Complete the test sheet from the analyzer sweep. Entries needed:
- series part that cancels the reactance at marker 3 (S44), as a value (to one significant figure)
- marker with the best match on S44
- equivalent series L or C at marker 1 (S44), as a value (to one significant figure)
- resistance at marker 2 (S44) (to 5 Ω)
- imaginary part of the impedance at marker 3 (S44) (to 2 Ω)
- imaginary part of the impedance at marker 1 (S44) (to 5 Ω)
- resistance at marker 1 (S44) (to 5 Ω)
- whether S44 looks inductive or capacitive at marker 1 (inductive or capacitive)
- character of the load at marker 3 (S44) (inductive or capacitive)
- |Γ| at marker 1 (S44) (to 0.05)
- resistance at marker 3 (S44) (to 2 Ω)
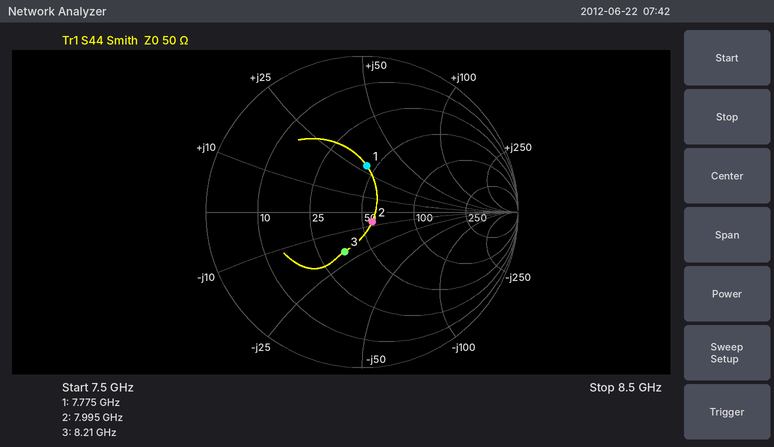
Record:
400 pH
marker 2
600 pH
55 Ω
-20 Ω
+30 Ω
45 Ω
inductive
capacitive
0.30
36 Ω
